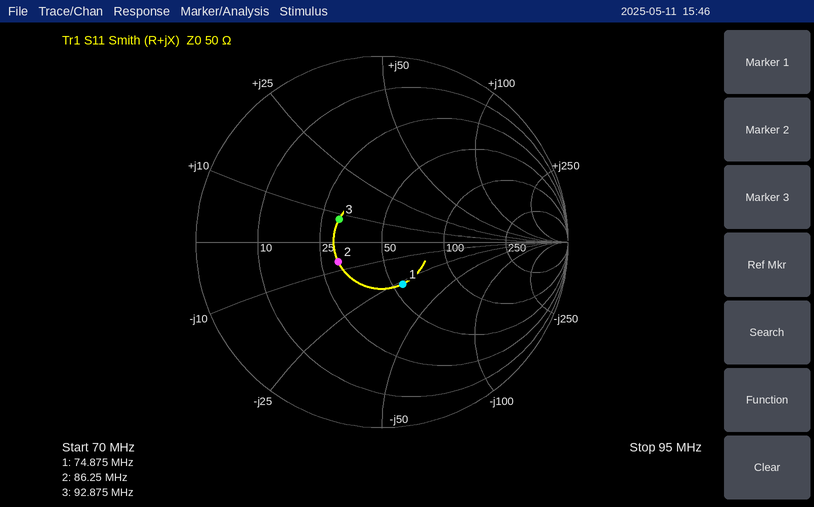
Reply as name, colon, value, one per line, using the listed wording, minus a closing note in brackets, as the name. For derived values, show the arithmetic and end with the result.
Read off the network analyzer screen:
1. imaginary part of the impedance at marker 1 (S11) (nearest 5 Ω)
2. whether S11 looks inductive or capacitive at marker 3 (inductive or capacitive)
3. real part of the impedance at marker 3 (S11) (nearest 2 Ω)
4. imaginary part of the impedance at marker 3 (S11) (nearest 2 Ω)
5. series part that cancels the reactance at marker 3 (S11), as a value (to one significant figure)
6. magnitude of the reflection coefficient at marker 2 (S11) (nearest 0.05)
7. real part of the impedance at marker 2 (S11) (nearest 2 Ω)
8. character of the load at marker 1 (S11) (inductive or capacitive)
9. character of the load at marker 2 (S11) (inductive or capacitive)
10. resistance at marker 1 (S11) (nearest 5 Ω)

imaginary part of the impedance at marker 1 (S11): -25 Ω
whether S11 looks inductive or capacitive at marker 3: inductive
real part of the impedance at marker 3 (S11): 30 Ω
imaginary part of the impedance at marker 3 (S11): +8 Ω
series part that cancels the reactance at marker 3 (S11), as a value: C = 1/(2π × 92.875 MHz × 8 Ω) ≈ 214 pF, so 200 pF to one significant figure
magnitude of the reflection coefficient at marker 2 (S11): 0.25
real part of the impedance at marker 2 (S11): 30 Ω
character of the load at marker 1 (S11): capacitive
character of the load at marker 2 (S11): capacitive
resistance at marker 1 (S11): 55 Ω
